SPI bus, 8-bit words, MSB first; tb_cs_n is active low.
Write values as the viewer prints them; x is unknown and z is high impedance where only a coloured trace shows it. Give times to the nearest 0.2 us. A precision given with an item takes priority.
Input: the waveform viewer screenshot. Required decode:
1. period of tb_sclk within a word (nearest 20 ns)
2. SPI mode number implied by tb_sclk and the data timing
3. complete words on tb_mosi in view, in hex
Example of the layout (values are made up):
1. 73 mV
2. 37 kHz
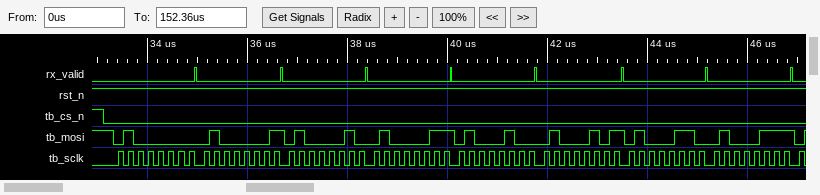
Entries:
1. 200 ns
2. 0
3. 40, 41, 42, 43, 44, 45, 46, 47
